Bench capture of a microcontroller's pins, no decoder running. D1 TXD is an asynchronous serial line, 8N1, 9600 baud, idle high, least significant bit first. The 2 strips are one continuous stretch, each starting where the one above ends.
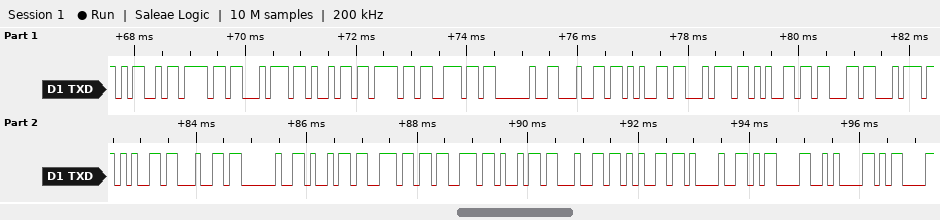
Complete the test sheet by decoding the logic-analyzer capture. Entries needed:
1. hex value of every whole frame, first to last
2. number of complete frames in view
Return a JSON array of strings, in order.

["0x4D 0x6F 0x74 0x69 0x6F 0x6E 0x20 0x64 0x65 0x74 0x65 0x63 0x74 0x65 0x64 0x20 0x69 0x6E 0x73 0x69 0x64 0x65 0x21 0x0D 0x0A 0x0D", "26"]
